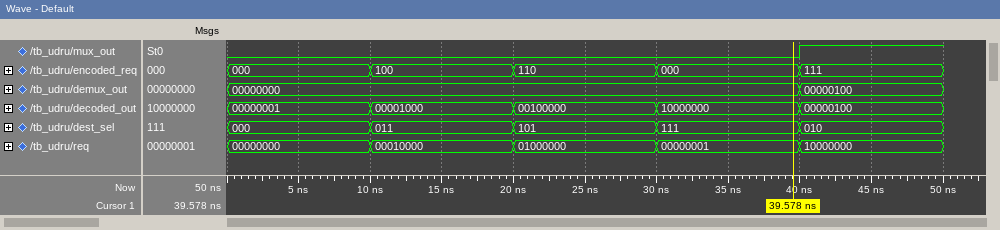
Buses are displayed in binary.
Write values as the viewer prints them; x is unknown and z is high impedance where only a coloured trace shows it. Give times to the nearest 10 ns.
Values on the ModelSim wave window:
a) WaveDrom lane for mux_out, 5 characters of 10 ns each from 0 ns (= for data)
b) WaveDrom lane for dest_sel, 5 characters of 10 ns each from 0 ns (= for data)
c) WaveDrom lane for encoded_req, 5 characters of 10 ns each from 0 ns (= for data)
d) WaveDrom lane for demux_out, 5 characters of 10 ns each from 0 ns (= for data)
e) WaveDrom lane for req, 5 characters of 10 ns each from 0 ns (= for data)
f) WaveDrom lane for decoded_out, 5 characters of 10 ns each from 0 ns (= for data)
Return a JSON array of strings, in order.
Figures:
["{name: 'mux_out', wave: '0...1'}", "{name: 'dest_sel', wave: '=====', data: '000 011 101 111 010'}", "{name: 'encoded_req', wave: '=====', data: '000 100 110 000 111'}", "{name: 'demux_out', wave: '=...=', data: '00000000 00000100'}", "{name: 'req', wave: '=====', data: '00000000 00010000 01000000 00000001 10000000'}", "{name: 'decoded_out', wave: '=====', data: '00000001 00001000 00100000 10000000 00000100'}"]
